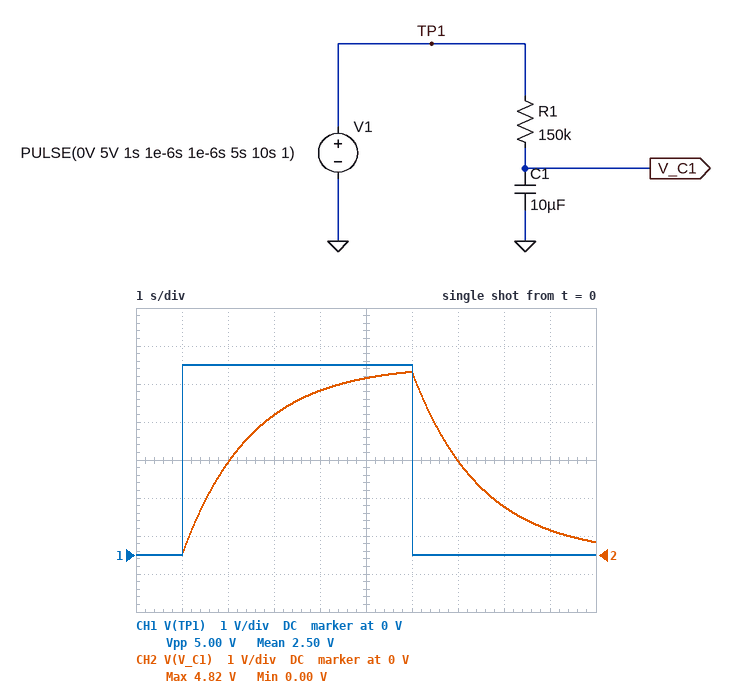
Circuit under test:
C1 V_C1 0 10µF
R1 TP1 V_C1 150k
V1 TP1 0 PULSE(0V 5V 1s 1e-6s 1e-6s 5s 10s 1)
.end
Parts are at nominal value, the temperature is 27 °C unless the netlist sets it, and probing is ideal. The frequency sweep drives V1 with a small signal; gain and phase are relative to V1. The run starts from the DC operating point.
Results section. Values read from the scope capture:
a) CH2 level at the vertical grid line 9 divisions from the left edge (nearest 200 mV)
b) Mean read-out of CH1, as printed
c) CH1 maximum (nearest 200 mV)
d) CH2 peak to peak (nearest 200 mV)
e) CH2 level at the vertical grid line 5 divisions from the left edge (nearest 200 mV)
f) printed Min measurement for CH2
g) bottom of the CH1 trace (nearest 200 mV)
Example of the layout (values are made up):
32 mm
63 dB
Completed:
600 mV
2.50 V
5.0 V
4.8 V
4.6 V
0.00 V
0 V
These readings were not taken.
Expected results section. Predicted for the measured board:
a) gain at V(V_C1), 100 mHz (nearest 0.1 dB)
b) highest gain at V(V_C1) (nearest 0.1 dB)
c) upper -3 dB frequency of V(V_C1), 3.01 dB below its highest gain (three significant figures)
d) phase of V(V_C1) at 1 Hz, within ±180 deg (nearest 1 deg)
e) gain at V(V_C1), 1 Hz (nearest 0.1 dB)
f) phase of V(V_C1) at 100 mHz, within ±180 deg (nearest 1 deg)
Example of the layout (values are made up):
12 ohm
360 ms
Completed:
-2.8 dB
0 dB
106 mHz
-84 deg
-19.5 dB
-43 deg
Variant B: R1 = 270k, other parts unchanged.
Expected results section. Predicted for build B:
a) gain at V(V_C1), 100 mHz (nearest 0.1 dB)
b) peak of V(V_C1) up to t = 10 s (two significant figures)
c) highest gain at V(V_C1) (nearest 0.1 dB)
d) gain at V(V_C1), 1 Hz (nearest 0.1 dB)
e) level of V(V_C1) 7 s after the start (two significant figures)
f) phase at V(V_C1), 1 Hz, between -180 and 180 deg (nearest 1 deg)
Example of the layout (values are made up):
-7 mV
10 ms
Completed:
-5.9 dB
4.2 V
0 dB
-24.6 dB
2.9 V
-87 deg
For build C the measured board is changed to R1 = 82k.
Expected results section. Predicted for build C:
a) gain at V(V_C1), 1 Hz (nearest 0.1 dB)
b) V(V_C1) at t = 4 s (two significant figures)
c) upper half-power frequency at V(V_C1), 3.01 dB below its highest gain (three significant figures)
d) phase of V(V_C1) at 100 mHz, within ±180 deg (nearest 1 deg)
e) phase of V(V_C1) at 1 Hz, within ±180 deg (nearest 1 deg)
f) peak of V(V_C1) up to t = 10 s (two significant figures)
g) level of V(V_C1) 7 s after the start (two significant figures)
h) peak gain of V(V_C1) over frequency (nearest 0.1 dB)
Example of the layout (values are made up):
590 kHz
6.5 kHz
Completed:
-14.4 dB
4.9 V
194 mHz
-27 deg
-79 deg
5.0 V
1.5 V
0 dB
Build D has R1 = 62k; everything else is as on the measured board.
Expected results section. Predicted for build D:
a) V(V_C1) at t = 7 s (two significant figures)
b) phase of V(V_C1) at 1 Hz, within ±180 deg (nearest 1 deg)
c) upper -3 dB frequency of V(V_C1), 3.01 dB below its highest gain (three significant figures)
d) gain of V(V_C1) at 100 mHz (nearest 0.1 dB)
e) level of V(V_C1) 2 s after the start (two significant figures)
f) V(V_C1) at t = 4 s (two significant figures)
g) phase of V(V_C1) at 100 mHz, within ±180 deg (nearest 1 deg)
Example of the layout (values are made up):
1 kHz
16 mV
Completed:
1.0 V
-76 deg
257 mHz
-0.6 dB
4.0 V
5.0 V
-21 deg
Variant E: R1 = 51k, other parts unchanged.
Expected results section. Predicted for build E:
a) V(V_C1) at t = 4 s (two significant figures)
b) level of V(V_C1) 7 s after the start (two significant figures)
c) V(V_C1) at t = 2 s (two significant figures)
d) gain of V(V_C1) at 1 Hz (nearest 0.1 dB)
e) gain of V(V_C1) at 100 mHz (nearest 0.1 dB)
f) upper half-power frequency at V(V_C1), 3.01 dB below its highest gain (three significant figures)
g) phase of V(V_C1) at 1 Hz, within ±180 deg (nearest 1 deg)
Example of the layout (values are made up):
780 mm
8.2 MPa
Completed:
5.0 V
700 mV
4.3 V
-10.5 dB
-0.4 dB
312 mHz
-73 deg
